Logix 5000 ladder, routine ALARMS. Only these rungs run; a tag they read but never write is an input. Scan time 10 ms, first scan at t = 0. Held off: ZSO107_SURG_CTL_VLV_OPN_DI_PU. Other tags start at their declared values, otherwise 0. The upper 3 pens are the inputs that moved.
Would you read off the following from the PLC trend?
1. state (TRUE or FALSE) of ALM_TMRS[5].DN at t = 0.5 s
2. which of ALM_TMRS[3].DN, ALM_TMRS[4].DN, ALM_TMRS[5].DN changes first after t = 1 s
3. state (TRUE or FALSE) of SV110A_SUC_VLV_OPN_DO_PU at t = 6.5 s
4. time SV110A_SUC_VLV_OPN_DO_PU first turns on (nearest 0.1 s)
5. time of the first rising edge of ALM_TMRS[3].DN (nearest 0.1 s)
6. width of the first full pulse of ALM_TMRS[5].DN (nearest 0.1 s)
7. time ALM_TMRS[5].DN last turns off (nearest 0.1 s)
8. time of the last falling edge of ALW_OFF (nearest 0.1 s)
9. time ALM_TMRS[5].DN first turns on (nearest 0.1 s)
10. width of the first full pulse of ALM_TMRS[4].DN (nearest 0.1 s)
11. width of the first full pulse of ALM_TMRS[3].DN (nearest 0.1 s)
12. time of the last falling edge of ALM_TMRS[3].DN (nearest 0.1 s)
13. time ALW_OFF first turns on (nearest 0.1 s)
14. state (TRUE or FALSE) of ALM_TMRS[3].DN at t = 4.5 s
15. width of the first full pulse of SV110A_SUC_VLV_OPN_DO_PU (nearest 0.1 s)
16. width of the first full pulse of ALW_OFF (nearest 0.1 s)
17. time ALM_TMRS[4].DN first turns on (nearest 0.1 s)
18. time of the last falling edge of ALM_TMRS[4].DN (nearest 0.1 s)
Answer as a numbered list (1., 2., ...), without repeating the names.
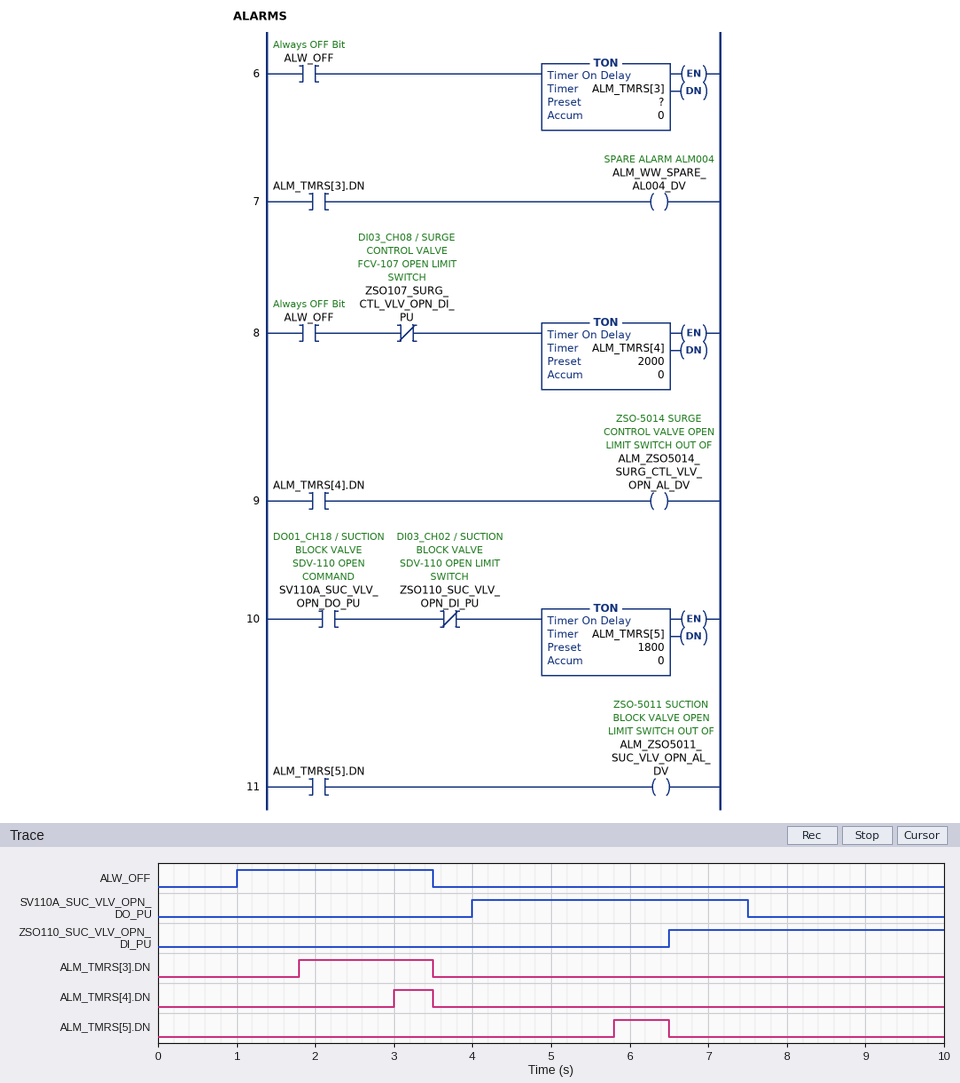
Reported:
1. FALSE
2. ALM_TMRS[3].DN
3. TRUE
4. 4.0 s
5. 1.8 s
6. 0.7 s
7. 6.5 s
8. 3.5 s
9. 5.8 s
10. 0.5 s
11. 1.7 s
12. 3.5 s
13. 1.0 s
14. FALSE
15. 3.5 s
16. 2.5 s
17. 3.0 s
18. 3.5 s
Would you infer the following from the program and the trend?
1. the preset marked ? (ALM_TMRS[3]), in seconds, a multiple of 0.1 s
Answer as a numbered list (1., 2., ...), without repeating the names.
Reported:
1. 0.8 s
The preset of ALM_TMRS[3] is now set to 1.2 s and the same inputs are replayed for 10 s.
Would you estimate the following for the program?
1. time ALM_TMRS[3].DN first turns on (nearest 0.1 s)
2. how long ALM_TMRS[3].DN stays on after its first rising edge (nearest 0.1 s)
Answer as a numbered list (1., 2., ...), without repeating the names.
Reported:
1. 2.2 s
2. 1.3 s
